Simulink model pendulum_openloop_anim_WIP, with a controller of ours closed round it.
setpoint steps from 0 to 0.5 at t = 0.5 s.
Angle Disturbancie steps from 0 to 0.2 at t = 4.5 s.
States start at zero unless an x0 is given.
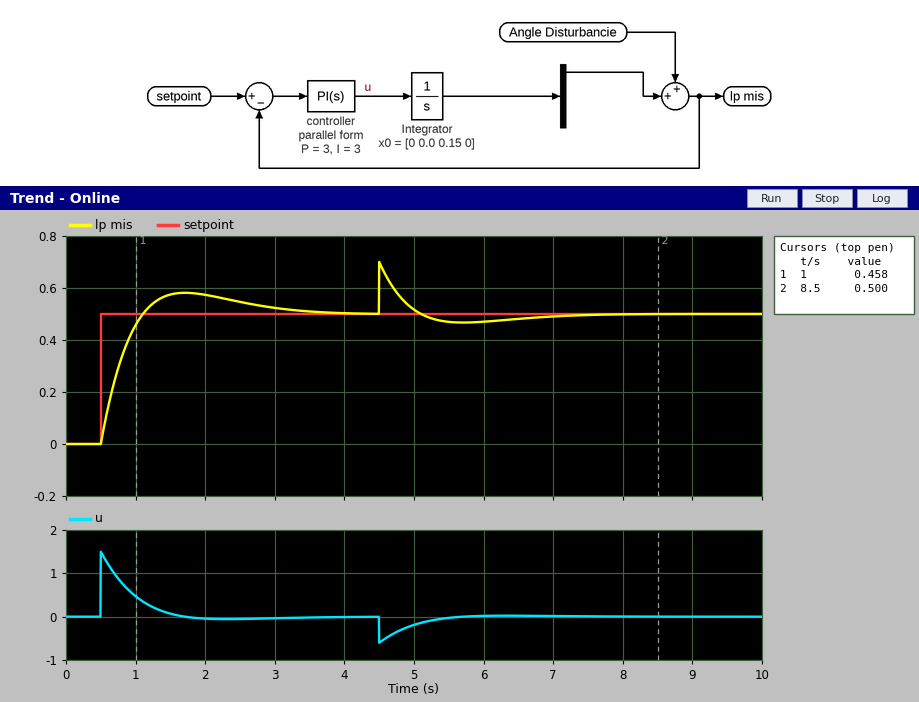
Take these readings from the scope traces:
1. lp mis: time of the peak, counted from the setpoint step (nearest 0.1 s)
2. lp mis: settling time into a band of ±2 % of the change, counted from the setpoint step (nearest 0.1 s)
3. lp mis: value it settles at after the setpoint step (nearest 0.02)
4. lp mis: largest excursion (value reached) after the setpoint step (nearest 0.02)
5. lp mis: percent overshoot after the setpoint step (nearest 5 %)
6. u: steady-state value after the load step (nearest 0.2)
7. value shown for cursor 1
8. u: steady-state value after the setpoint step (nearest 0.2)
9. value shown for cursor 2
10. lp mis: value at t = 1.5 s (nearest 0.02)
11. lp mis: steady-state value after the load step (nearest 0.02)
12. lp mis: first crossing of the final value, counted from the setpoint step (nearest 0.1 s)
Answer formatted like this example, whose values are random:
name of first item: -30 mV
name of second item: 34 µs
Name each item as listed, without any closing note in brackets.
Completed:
lp mis: time of the peak, counted from the setpoint step: 1.2 s
lp mis: settling time into a band of ±2 % of the change, counted from the setpoint step: 3.0 s
lp mis: value it settles at after the setpoint step: 0.50
lp mis: largest excursion (value reached) after the setpoint step: 0.58
lp mis: percent overshoot after the setpoint step: 15 %
u: steady-state value after the load step: 0.0
value shown for cursor 1: 0.458
u: steady-state value after the setpoint step: 0.0
value shown for cursor 2: 0.500
lp mis: value at t = 1.5 s: 0.58
lp mis: steady-state value after the load step: 0.50
lp mis: first crossing of the final value, counted from the setpoint step: 0.6 s
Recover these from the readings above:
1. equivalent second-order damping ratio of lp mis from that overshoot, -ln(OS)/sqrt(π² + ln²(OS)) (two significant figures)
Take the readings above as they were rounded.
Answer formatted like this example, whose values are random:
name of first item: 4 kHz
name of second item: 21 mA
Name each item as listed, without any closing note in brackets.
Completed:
equivalent second-order damping ratio of lp mis from that overshoot, -ln(OS)/sqrt(π² + ln²(OS)): 0.52
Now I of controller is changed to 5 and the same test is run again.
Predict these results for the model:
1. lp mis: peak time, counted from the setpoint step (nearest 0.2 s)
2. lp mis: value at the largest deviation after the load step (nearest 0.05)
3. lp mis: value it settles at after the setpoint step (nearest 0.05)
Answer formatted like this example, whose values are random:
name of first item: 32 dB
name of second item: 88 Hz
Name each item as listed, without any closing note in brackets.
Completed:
lp mis: peak time, counted from the setpoint step: 1.0 s
lp mis: value at the largest deviation after the load step: 0.70
lp mis: value it settles at after the setpoint step: 0.50
